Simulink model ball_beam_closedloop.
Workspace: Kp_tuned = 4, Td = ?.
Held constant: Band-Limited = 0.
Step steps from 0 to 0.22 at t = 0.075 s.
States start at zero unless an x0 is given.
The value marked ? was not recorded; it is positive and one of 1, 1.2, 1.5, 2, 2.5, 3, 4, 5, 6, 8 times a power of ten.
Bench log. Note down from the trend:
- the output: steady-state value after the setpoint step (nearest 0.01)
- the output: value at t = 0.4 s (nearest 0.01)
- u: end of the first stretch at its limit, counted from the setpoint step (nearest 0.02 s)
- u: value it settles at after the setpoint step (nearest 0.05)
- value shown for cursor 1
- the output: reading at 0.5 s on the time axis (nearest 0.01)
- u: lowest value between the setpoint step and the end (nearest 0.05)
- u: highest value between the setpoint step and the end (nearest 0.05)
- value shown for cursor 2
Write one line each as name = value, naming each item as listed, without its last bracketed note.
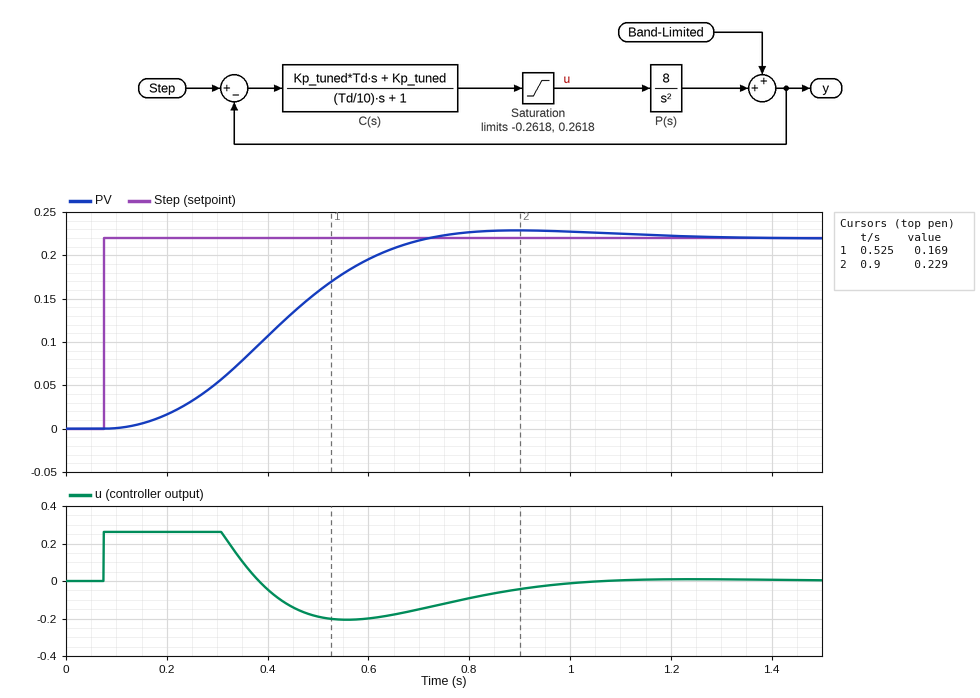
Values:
the output: steady-state value after the setpoint step = 0.22
the output: value at t = 0.4 s = 0.11
u: end of the first stretch at its limit, counted from the setpoint step = 0.24 s
u: value it settles at after the setpoint step = 0.00
value shown for cursor 1 = 0.169
the output: reading at 0.5 s on the time axis = 0.16
u: lowest value between the setpoint step and the end = -0.20
u: highest value between the setpoint step and the end = 0.25
value shown for cursor 2 = 0.229
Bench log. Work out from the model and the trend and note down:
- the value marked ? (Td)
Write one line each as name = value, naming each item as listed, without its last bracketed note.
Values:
the value marked ? = 0.25
